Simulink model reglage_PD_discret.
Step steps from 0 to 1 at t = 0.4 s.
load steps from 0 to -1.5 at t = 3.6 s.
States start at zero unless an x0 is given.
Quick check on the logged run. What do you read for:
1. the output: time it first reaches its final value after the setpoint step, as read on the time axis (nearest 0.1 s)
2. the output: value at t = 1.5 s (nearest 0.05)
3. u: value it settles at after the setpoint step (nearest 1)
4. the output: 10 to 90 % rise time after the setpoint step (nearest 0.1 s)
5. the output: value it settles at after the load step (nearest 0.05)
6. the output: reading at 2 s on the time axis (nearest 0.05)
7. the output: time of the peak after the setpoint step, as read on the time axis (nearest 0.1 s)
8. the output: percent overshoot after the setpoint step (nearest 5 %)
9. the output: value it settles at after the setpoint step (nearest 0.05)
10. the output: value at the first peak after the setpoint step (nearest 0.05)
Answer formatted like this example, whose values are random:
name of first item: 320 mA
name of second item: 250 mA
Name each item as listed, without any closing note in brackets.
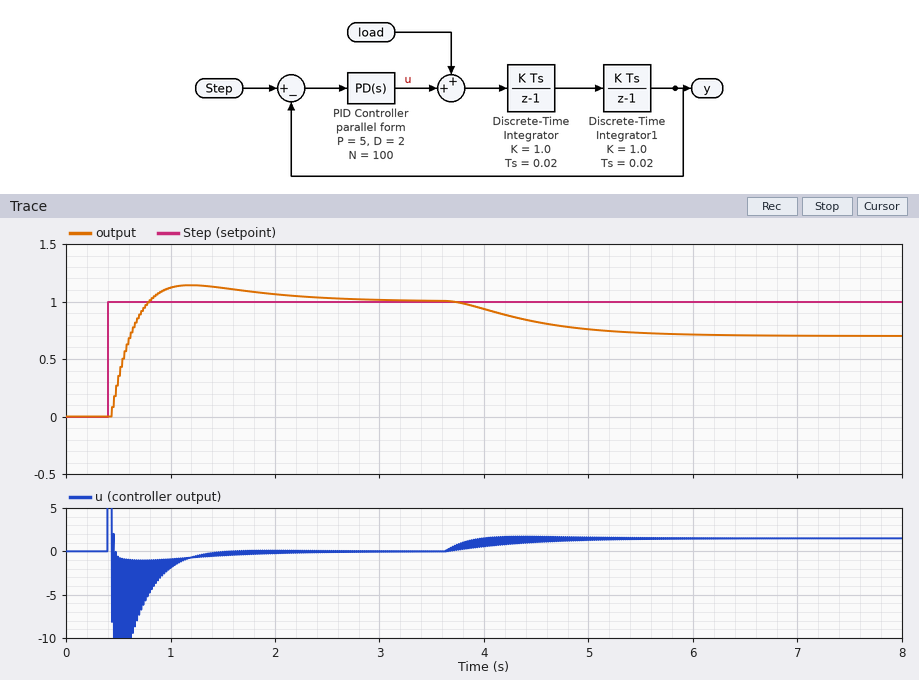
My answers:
the output: time it first reaches its final value after the setpoint step, as read on the time axis: 0.8 s
the output: value at t = 1.5 s: 1.10
u: value it settles at after the setpoint step: 0
the output: 10 to 90 % rise time after the setpoint step: 0.3 s
the output: value it settles at after the load step: 0.70
the output: reading at 2 s on the time axis: 1.05
the output: time of the peak after the setpoint step, as read on the time axis: 1.2 s
the output: percent overshoot after the setpoint step: 15 %
the output: value it settles at after the setpoint step: 1.00
the output: value at the first peak after the setpoint step: 1.15
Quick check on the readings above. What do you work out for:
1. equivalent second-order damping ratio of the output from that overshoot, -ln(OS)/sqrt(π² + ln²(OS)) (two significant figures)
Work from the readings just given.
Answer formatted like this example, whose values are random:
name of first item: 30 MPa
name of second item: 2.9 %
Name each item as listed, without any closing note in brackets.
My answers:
equivalent second-order damping ratio of the output from that overshoot, -ln(OS)/sqrt(π² + ln²(OS)): 0.52
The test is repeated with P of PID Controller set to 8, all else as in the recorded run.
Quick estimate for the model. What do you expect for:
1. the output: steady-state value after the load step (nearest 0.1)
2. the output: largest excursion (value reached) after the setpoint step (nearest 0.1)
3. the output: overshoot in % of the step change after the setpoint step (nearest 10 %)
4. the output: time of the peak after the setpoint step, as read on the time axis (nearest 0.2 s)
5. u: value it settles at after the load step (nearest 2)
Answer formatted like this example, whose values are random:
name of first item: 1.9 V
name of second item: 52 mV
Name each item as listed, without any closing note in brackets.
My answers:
the output: steady-state value after the load step: 0.8
the output: largest excursion (value reached) after the setpoint step: 1.2
the output: overshoot in % of the step change after the setpoint step: 20 %
the output: time of the peak after the setpoint step, as read on the time axis: 1.0 s
u: value it settles at after the load step: 2
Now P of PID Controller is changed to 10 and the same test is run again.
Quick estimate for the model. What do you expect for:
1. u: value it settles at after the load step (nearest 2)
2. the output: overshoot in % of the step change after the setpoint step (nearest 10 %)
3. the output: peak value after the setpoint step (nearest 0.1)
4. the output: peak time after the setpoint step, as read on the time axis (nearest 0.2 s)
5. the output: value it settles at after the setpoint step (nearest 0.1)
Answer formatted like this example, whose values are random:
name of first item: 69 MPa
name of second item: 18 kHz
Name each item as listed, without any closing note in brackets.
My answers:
u: value it settles at after the load step: 2
the output: overshoot in % of the step change after the setpoint step: 20 %
the output: peak value after the setpoint step: 1.2
the output: peak time after the setpoint step, as read on the time axis: 1.0 s
the output: value it settles at after the setpoint step: 1.0
